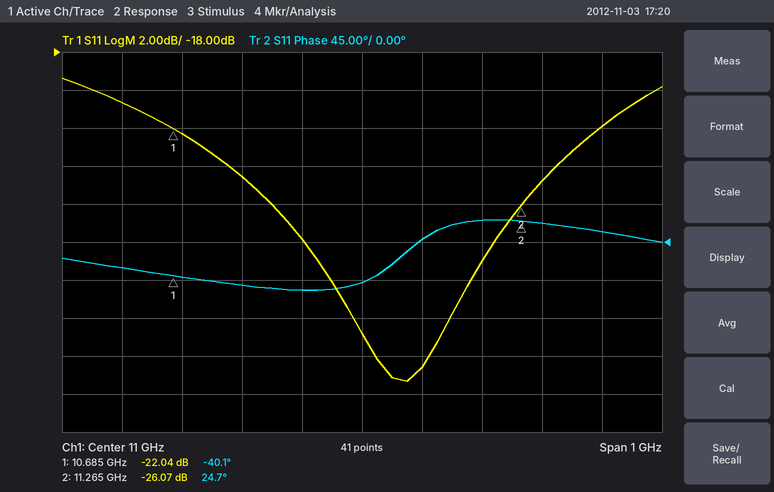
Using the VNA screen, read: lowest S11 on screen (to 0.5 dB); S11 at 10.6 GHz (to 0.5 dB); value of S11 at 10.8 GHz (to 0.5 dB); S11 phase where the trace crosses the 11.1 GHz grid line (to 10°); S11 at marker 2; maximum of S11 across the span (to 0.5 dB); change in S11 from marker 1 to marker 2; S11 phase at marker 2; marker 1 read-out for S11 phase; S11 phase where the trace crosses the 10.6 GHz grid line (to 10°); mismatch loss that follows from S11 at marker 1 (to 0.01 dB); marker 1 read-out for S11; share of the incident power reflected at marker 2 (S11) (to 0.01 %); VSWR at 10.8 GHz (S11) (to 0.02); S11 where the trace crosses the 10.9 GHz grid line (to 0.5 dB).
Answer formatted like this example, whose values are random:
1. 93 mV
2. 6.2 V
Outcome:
1. -35.5 dB
2. -20.5 dB
3. -24.5 dB
4. 0°
5. -26.07 dB
6. -19.5 dB
7. -4.03 dB
8. 24.7°
9. -40.1°
10. -30°
11. 0.03 dB
12. -22.04 dB
13. 0.25 %
14. 1.12
15. -28.0 dB
